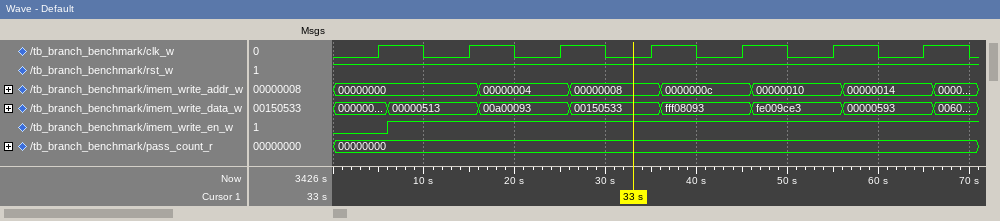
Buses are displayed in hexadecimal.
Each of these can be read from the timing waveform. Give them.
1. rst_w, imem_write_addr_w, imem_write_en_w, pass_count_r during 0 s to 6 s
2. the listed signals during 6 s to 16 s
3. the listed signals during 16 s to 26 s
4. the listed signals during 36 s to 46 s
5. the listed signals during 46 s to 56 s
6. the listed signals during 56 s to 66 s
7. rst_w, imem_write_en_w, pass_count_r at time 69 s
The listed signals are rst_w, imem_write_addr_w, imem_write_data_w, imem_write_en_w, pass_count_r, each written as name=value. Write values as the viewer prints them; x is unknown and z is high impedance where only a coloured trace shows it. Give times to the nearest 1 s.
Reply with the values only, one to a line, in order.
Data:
rst_w=1, imem_write_addr_w=00000000, imem_write_en_w=0, pass_count_r=00000000
rst_w=1, imem_write_addr_w=00000000, imem_write_data_w=00000513, imem_write_en_w=1, pass_count_r=00000000
rst_w=1, imem_write_addr_w=00000004, imem_write_data_w=00a00093, imem_write_en_w=1, pass_count_r=00000000
rst_w=1, imem_write_addr_w=0000000c, imem_write_data_w=fff08093, imem_write_en_w=1, pass_count_r=00000000
rst_w=1, imem_write_addr_w=00000010, imem_write_data_w=fe009ce3, imem_write_en_w=1, pass_count_r=00000000
rst_w=1, imem_write_addr_w=00000014, imem_write_data_w=00000593, imem_write_en_w=1, pass_count_r=00000000
rst_w=1, imem_write_en_w=1, pass_count_r=00000000
